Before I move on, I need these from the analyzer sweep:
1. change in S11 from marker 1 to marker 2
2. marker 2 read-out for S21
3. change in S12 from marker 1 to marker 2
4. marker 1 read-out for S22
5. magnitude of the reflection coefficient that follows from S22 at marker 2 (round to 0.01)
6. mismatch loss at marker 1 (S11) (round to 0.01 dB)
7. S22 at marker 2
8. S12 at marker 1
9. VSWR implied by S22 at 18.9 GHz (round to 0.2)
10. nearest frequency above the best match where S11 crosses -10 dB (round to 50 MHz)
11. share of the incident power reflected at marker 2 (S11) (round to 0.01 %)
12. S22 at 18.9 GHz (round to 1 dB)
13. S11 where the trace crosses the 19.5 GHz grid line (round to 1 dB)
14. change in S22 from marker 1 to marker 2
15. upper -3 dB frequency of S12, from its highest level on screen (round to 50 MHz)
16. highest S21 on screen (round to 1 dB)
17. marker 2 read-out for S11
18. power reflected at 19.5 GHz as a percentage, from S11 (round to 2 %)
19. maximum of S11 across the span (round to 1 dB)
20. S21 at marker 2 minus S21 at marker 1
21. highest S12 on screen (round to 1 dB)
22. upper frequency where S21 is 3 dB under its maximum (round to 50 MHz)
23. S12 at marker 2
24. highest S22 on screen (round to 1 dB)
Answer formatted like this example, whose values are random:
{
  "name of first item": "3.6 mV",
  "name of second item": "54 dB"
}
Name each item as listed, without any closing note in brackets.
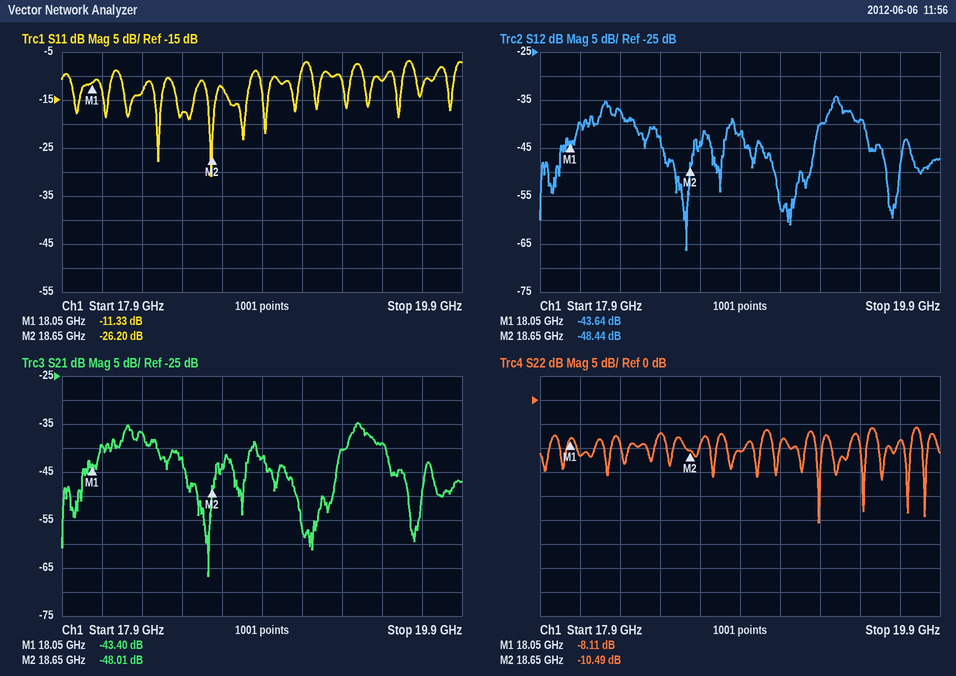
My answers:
{
  "change in S11 from marker 1 to marker 2": "-14.87 dB",
  "marker 2 read-out for S21": "-48.01 dB",
  "change in S12 from marker 1 to marker 2": "-4.80 dB",
  "marker 1 read-out for S22": "-8.11 dB",
  "magnitude of the reflection coefficient that follows from S22 at marker 2": "0.30",
  "mismatch loss at marker 1 (S11)": "0.33 dB",
  "S22 at marker 2": "-10.49 dB",
  "S12 at marker 1": "-43.64 dB",
  "VSWR implied by S22 at 18.9 GHz": "1.8",
  "nearest frequency above the best match where S11 crosses -10 dB": "18.85 GHz",
  "share of the incident power reflected at marker 2 (S11)": "0.24 %",
  "S22 at 18.9 GHz": "-11 dB",
  "S11 where the trace crosses the 19.5 GHz grid line": "-11 dB",
  "change in S22 from marker 1 to marker 2": "-2.38 dB",
  "upper -3 dB frequency of S12, from its highest level on screen": "19.40 GHz",
  "highest S21 on screen": "-35 dB",
  "marker 2 read-out for S11": "-26.20 dB",
  "power reflected at 19.5 GHz as a percentage, from S11": "8 %",
  "maximum of S11 across the span": "-7 dB",
  "S21 at marker 2 minus S21 at marker 1": "-4.61 dB",
  "highest S12 on screen": "-34 dB",
  "upper frequency where S21 is 3 dB under its maximum": "19.45 GHz",
  "S12 at marker 2": "-48.44 dB",
  "highest S22 on screen": "-6 dB"
}
